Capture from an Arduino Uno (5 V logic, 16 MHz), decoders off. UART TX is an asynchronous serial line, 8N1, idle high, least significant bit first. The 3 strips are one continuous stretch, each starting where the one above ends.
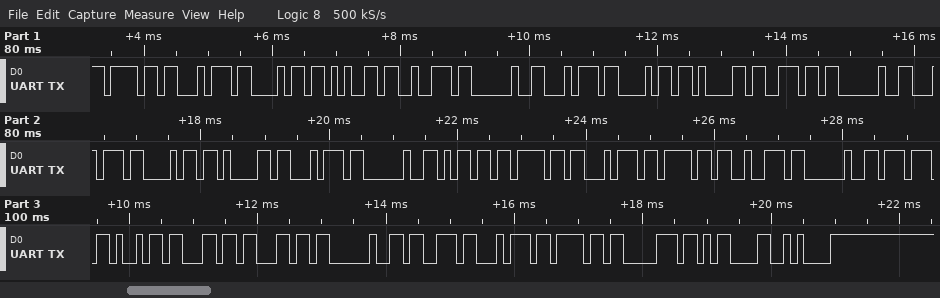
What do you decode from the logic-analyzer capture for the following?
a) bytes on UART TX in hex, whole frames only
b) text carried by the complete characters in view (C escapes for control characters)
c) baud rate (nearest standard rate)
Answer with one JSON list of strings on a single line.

["6F 74 68 65 72 20 74 68 61 6E 20 74 68 61 74 20 6D 6F 74 6F 72 20 77 69 6C 6C 20 73 74 6F 70 0D 0A", "\"other than that motor will stop\\r\\n\"", "9600 baud"]
